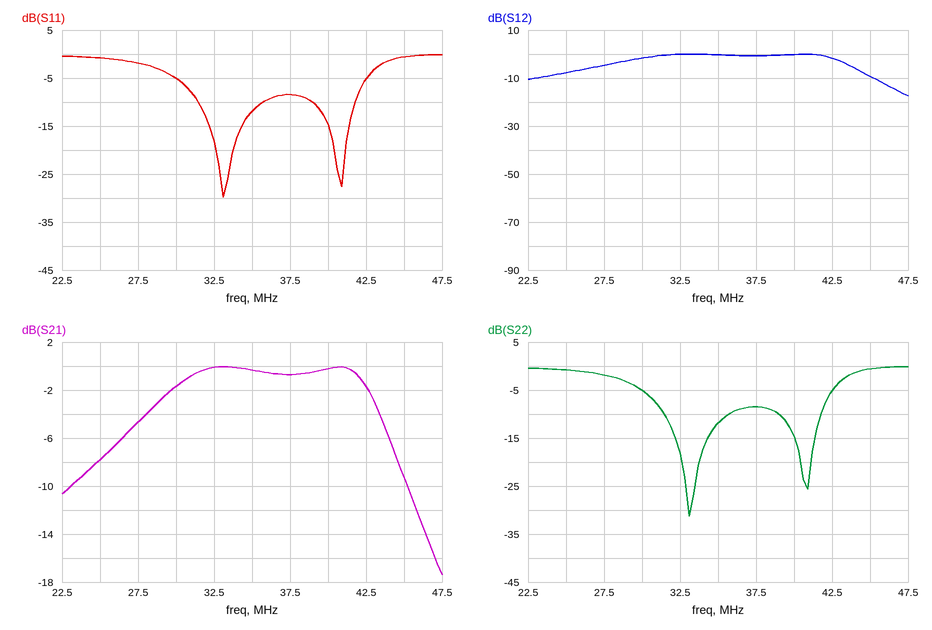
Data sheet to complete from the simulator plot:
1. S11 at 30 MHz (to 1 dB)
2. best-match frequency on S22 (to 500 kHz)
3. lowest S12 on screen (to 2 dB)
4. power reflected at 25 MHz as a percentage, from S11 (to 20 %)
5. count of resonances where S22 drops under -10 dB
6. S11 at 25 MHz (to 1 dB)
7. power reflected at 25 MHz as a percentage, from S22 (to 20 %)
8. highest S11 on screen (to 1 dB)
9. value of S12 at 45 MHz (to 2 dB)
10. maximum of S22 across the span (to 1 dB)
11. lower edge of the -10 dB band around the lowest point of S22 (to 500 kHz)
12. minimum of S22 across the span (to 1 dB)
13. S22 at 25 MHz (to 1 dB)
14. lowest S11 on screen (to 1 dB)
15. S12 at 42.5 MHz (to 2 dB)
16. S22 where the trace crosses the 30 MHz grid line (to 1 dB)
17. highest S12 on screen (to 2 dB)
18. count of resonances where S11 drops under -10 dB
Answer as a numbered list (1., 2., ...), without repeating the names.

1. -5 dB
2. 33.0 MHz
3. -18 dB
4. 80 %
5. 2
6. -1 dB
7. 80 %
8. 0 dB
9. -10 dB
10. 0 dB
11. 31.5 MHz
12. -31 dB
13. -1 dB
14. -30 dB
15. -2 dB
16. -5 dB
17. 0 dB
18. 2
